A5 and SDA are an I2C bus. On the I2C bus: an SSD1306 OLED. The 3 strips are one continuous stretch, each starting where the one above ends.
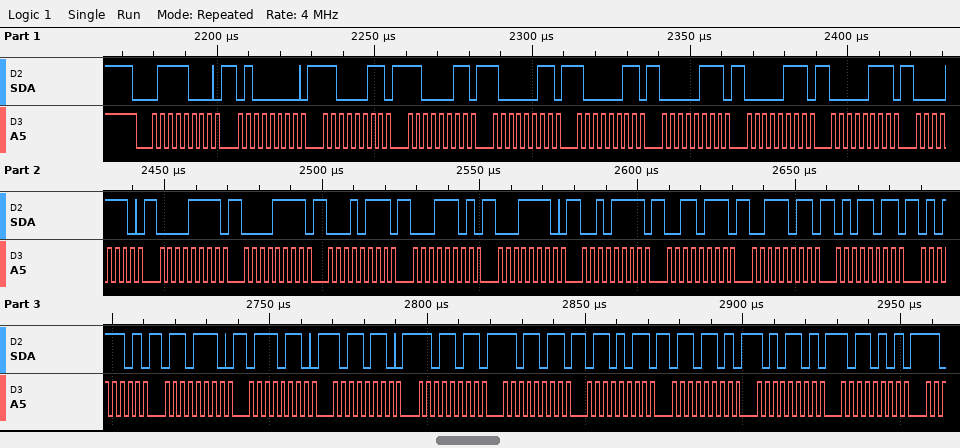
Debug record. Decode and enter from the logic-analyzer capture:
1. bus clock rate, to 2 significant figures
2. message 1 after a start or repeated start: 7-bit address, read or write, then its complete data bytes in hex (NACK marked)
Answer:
400 kHz
0x3C write: 40 C3 C3 83 83 07 07 07 0E 0F 0F 17 1D 1E 2F 37 3B 5B 5D 6E 76 B6 DB DB 6B 6D AD B5
